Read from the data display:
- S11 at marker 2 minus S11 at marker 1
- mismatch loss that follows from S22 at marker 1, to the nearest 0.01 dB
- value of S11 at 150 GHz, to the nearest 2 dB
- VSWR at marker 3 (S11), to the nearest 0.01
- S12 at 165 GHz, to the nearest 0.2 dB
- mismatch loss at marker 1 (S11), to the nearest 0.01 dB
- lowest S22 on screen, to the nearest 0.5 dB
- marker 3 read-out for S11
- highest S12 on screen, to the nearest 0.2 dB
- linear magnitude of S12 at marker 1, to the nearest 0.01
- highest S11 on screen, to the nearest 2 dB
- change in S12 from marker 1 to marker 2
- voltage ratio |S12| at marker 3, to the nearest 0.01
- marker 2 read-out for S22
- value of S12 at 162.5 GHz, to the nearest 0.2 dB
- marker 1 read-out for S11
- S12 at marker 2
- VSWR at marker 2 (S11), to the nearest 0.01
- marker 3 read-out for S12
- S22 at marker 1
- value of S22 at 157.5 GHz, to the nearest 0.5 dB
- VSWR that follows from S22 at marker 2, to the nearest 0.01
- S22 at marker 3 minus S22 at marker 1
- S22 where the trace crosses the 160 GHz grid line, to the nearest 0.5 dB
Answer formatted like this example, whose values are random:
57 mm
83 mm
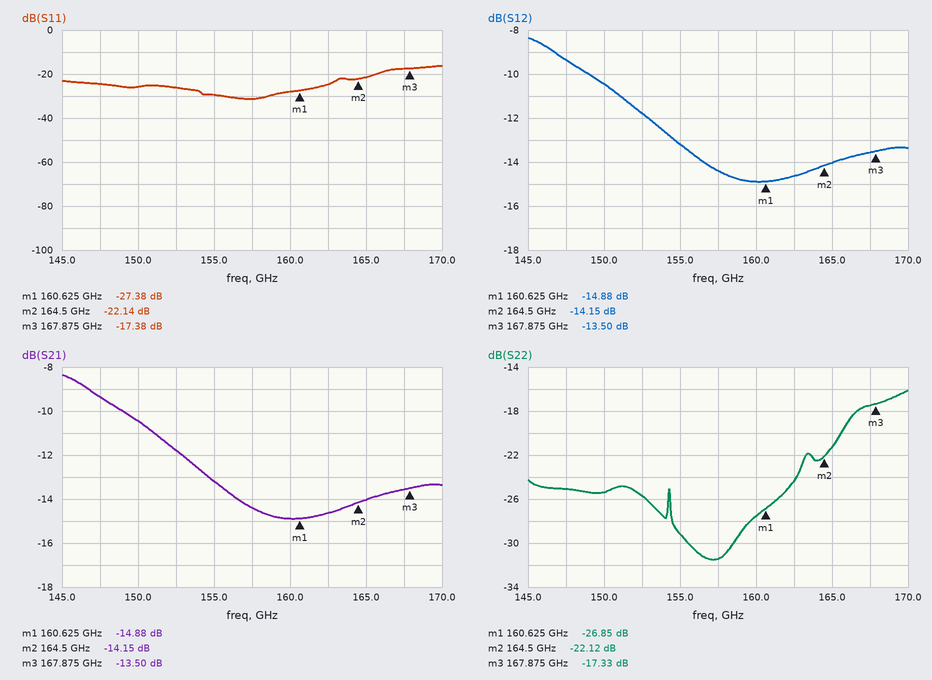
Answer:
5.24 dB
0.01 dB
-26 dB
1.31
-14.0 dB
0.01 dB
-31.5 dB
-17.38 dB
-8.4 dB
0.18
-16 dB
0.73 dB
0.21
-22.12 dB
-14.6 dB
-27.38 dB
-14.15 dB
1.17
-13.50 dB
-26.85 dB
-31.5 dB
1.17
9.52 dB
-27.5 dB
